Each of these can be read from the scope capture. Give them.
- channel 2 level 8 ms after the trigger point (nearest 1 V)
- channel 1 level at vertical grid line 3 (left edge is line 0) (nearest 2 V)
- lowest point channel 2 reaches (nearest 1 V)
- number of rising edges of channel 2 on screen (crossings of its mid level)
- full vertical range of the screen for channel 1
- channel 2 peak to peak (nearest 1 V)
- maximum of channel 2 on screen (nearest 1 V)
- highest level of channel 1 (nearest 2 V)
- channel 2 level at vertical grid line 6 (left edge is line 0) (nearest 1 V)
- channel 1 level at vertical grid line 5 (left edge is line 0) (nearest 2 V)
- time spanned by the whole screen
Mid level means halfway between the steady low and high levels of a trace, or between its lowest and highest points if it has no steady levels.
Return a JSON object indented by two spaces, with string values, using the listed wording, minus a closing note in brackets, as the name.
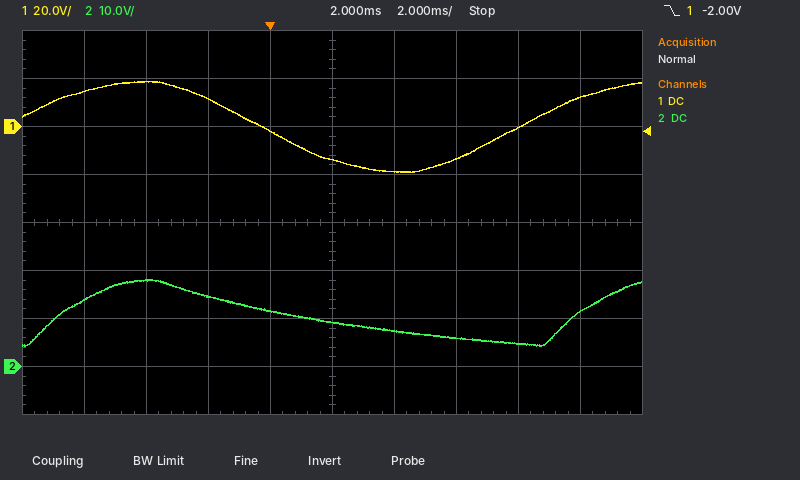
{
  "channel 2 level 8 ms after the trigger point": "5 V",
  "channel 1 level at vertical grid line 3 (left edge is line 0)": "12 V",
  "lowest point channel 2 reaches": "4 V",
  "number of rising edges of channel 2 on screen": "2",
  "full vertical range of the screen for channel 1": "160 V",
  "channel 2 peak to peak": "14 V",
  "maximum of channel 2 on screen": "18 V",
  "highest level of channel 1": "18 V",
  "channel 2 level at vertical grid line 6 (left edge is line 0)": "7 V",
  "channel 1 level at vertical grid line 5 (left edge is line 0)": "-14 V",
  "time spanned by the whole screen": "20 ms"
}
